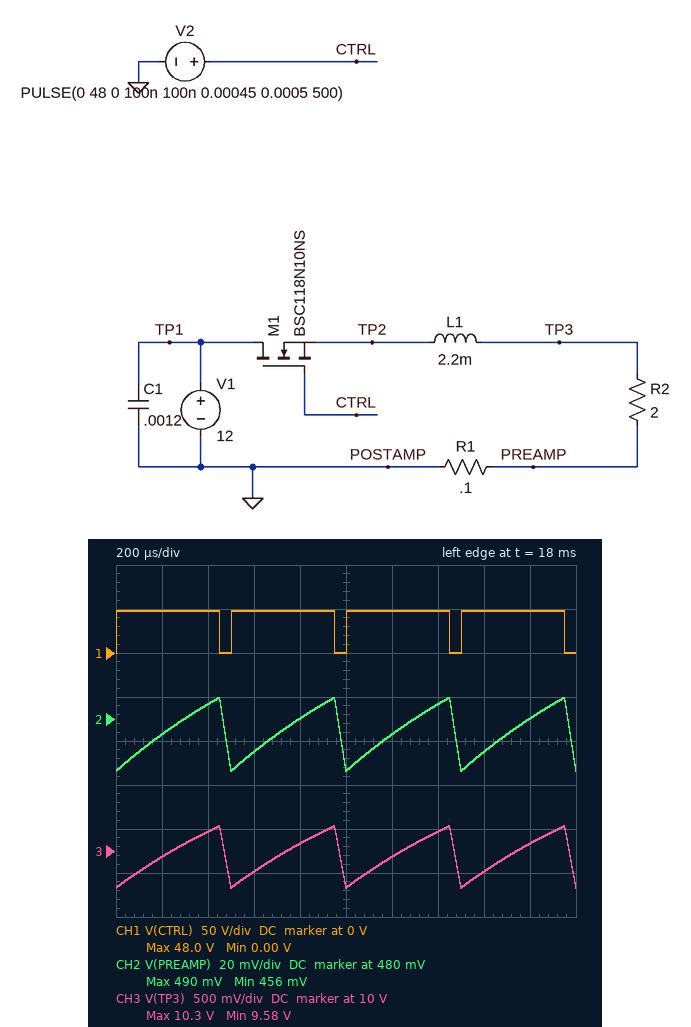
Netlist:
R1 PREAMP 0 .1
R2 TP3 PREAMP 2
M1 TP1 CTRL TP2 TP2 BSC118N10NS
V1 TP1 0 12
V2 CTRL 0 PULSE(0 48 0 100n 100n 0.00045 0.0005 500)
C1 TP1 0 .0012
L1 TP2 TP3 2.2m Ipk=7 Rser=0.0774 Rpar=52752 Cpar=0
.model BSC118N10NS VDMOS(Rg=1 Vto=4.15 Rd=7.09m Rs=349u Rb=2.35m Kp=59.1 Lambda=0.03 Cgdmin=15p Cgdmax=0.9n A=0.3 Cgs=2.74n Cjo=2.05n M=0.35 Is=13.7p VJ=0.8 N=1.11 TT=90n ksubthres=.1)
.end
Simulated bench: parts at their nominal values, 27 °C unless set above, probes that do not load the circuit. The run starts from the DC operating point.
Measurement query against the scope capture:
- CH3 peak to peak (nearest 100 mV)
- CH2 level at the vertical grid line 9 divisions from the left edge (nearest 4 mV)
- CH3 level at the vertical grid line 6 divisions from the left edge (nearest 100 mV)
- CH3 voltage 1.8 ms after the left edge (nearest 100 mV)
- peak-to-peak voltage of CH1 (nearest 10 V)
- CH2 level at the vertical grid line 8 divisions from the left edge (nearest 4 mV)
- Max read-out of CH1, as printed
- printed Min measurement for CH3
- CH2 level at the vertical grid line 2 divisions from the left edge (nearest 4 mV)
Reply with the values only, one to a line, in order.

700 mV
480 mV
9.9 V
10.1 V
50 V
464 mV
48.0 V
9.58 V
488 mV
